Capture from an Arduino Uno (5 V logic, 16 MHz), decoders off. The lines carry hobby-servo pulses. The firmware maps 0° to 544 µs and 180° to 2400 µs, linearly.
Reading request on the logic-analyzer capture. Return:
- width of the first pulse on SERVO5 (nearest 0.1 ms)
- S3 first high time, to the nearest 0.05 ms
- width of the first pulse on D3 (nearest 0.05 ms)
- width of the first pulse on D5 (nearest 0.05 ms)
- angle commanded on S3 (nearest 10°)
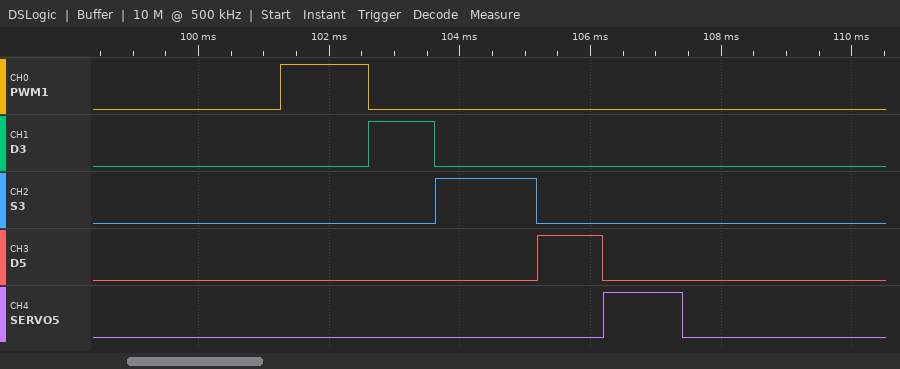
1.2 ms
1.55 ms
1.00 ms
1.00 ms
100°
